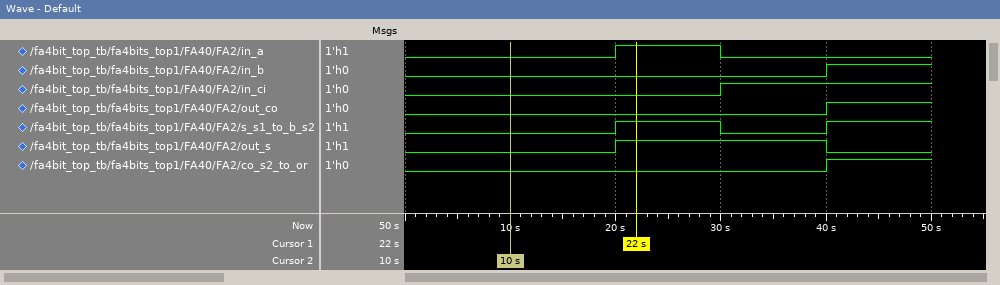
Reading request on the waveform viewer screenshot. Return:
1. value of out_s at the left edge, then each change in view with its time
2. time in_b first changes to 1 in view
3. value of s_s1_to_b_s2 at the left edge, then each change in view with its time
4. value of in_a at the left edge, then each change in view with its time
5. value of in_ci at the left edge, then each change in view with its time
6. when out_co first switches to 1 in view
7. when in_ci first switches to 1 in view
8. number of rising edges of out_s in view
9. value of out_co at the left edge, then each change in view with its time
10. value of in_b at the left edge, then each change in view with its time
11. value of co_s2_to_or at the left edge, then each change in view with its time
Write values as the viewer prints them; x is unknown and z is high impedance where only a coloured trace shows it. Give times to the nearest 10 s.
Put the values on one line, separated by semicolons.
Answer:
0, 1 at 20 s, 0 at 40 s; 40 s; 0, 1 at 20 s, 0 at 30 s, 1 at 40 s; 0, 1 at 20 s, 0 at 30 s; 0, 1 at 30 s; 40 s; 30 s; 1; 0, 1 at 40 s; 0, 1 at 40 s; 0, 1 at 40 s
